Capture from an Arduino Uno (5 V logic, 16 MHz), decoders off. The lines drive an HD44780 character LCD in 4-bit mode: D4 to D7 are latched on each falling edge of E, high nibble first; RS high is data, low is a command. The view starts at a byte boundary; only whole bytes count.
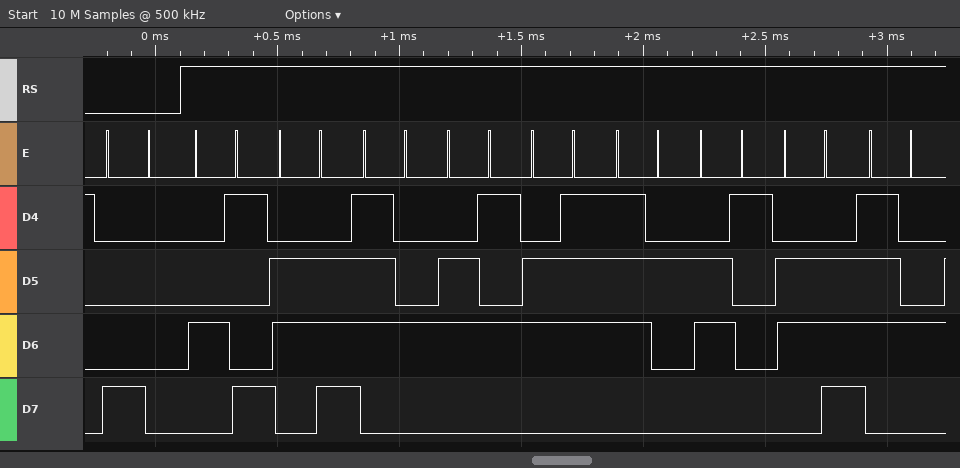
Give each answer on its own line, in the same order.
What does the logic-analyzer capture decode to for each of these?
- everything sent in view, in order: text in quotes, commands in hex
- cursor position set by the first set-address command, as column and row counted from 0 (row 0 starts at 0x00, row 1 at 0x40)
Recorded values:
0x80 "Integrant"
column 0, row 0
